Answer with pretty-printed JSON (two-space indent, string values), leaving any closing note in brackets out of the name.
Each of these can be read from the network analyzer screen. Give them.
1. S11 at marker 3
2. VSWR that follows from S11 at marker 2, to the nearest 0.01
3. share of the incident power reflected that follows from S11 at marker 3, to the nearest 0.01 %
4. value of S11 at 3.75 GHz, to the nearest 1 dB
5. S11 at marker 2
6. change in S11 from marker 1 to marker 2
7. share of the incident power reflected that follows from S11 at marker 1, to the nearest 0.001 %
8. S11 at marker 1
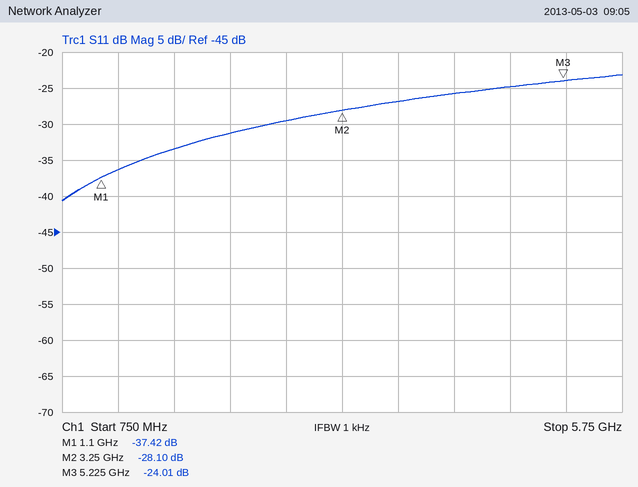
{
  "S11 at marker 3": "-24.01 dB",
  "VSWR that follows from S11 at marker 2, to the nearest 0.01": "1.08",
  "share of the incident power reflected that follows from S11 at marker 3, to the nearest 0.01 %": "0.40 %",
  "value of S11 at 3.75 GHz, to the nearest 1 dB": "-27 dB",
  "S11 at marker 2": "-28.10 dB",
  "change in S11 from marker 1 to marker 2": "9.32 dB",
  "share of the incident power reflected that follows from S11 at marker 1, to the nearest 0.001 %": "0.018 %",
  "S11 at marker 1": "-37.42 dB"
}
